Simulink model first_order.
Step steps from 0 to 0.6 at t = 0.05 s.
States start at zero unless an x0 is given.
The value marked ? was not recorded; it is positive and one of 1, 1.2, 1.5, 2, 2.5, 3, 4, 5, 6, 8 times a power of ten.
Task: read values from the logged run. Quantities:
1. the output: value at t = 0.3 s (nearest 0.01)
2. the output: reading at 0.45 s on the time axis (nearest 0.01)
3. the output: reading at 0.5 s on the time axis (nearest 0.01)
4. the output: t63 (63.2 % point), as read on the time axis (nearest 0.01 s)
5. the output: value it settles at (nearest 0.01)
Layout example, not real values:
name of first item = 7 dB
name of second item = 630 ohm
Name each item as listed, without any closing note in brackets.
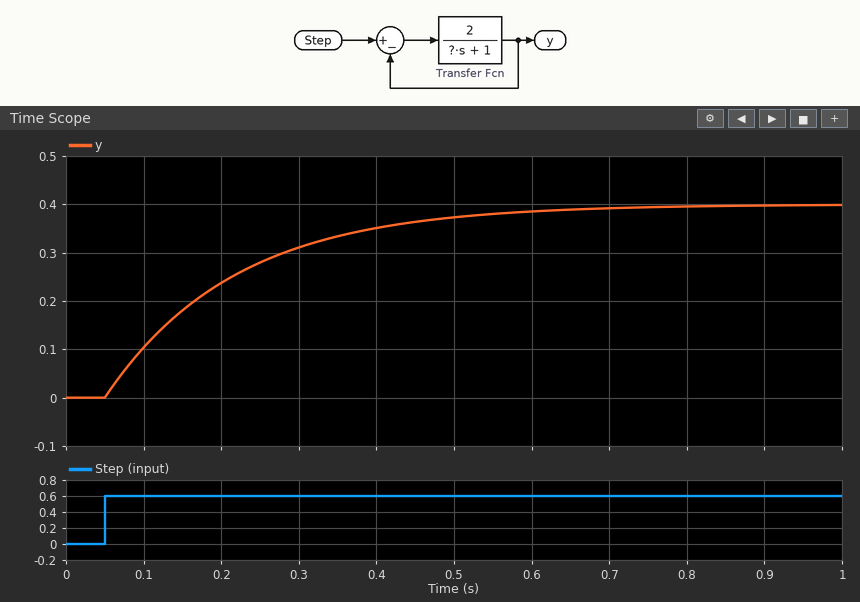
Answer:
the output: value at t = 0.3 s = 0.31
the output: reading at 0.45 s on the time axis = 0.36
the output: reading at 0.5 s on the time axis = 0.37
the output: t63 (63.2 % point), as read on the time axis = 0.22 s
the output: value it settles at = 0.40
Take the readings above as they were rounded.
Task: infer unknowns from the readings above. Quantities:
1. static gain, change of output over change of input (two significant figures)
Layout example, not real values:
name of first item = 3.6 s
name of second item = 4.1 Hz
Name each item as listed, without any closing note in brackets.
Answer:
static gain, change of output over change of input = 0.67
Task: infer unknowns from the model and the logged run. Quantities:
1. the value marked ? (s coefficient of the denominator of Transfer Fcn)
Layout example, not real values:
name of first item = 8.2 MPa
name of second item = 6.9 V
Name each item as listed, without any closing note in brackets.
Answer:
the value marked ? = 0.5
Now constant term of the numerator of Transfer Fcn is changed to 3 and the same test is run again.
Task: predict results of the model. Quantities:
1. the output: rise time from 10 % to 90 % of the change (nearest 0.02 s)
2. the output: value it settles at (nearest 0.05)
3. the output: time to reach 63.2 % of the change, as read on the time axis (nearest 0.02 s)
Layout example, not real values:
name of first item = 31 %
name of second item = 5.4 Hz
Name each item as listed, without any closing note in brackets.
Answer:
the output: rise time from 10 % to 90 % of the change = 0.28 s
the output: value it settles at = 0.45
the output: time to reach 63.2 % of the change, as read on the time axis = 0.18 s
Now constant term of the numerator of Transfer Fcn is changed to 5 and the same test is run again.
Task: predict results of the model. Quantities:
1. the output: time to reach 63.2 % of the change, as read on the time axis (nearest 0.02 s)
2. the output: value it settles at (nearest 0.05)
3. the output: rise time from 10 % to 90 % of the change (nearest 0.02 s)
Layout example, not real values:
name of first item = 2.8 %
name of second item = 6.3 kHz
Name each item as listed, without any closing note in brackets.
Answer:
the output: time to reach 63.2 % of the change, as read on the time axis = 0.14 s
the output: value it settles at = 0.50
the output: rise time from 10 % to 90 % of the change = 0.18 s
